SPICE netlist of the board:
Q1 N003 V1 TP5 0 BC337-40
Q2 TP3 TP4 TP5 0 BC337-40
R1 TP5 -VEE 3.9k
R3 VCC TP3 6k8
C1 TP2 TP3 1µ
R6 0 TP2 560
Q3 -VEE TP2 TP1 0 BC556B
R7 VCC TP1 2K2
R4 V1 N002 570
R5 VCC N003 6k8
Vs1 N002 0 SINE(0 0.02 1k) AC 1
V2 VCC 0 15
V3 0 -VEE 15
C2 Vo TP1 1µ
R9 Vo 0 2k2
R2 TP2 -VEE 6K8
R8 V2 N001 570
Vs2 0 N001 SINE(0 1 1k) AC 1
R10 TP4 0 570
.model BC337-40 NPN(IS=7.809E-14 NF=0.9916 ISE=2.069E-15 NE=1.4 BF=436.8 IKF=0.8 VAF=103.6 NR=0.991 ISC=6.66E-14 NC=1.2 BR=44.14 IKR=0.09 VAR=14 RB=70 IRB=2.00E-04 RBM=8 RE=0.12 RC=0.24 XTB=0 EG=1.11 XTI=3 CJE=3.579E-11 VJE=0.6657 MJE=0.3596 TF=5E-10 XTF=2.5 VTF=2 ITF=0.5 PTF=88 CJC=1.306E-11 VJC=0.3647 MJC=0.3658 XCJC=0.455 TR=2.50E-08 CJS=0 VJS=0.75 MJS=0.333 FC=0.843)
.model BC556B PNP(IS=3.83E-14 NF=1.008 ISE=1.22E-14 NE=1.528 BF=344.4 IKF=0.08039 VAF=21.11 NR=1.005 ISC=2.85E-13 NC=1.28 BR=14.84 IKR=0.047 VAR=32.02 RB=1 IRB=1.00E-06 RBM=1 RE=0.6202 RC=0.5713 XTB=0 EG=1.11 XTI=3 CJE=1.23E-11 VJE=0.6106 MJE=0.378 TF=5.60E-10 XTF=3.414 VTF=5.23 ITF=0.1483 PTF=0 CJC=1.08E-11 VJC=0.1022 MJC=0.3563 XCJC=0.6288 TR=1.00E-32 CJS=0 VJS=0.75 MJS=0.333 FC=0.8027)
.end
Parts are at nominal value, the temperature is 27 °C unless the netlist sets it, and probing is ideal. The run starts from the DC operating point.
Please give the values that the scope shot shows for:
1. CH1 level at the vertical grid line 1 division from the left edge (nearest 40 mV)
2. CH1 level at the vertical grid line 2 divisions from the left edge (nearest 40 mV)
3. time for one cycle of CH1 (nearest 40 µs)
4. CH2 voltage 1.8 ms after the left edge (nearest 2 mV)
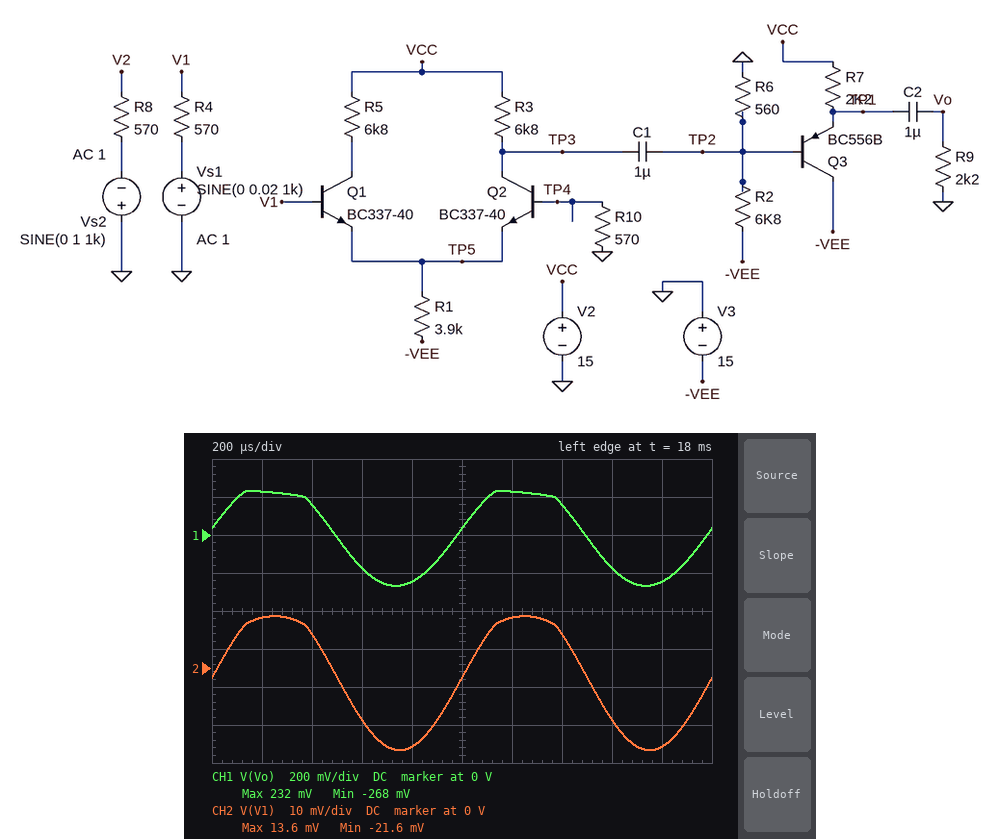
240 mV
160 mV
1.00 ms
-20 mV
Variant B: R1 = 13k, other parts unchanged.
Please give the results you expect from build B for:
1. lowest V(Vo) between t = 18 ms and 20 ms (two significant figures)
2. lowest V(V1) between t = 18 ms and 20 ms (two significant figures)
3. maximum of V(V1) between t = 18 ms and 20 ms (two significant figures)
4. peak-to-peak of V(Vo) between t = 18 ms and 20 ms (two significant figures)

-93 mV
-20 mV
19 mV
190 mV
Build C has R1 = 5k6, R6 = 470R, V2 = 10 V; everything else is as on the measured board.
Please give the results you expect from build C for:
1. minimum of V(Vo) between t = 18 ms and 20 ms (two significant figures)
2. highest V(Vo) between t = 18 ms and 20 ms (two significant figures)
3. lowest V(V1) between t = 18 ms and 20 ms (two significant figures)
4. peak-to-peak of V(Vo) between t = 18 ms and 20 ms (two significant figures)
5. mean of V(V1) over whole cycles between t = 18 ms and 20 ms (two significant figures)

-160 mV
130 mV
-21 mV
290 mV
-2.6 mV
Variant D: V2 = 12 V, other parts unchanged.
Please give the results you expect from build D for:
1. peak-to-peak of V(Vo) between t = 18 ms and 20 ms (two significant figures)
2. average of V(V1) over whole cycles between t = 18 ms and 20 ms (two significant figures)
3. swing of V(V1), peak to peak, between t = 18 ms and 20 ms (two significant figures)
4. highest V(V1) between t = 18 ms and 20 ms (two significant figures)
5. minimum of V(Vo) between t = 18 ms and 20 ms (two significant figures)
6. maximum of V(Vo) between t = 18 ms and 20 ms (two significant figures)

57 mV
-7.4 mV
26 mV
3.7 mV
-36 mV
21 mV
